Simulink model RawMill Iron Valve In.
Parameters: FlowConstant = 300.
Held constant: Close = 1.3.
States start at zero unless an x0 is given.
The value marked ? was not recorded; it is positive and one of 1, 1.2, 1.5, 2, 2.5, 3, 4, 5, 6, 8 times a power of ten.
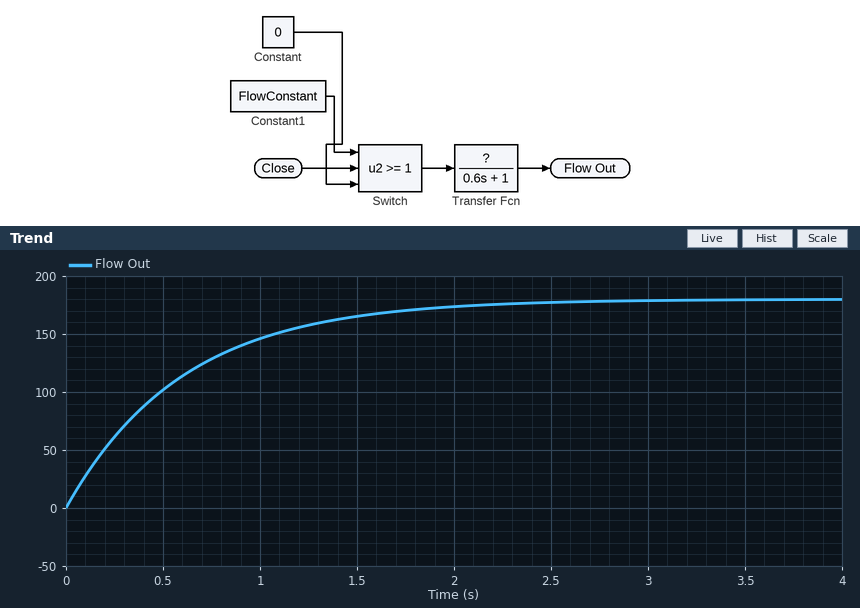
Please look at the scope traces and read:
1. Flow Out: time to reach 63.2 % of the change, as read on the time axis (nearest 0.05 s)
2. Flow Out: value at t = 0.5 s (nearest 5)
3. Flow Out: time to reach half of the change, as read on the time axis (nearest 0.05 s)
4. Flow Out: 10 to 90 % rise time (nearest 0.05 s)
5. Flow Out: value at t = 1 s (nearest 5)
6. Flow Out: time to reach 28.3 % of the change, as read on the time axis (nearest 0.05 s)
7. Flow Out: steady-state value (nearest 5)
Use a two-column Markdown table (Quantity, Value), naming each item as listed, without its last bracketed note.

| Quantity | Value |
|---|---|
| Flow Out: time to reach 63.2 % of the change, as read on the time axis | 0.60 s |
| Flow Out: value at t = 0.5 s | 100 |
| Flow Out: time to reach half of the change, as read on the time axis | 0.40 s |
| Flow Out: 10 to 90 % rise time | 1.30 s |
| Flow Out: value at t = 1 s | 145 |
| Flow Out: time to reach 28.3 % of the change, as read on the time axis | 0.20 s |
| Flow Out: steady-state value | 180 |
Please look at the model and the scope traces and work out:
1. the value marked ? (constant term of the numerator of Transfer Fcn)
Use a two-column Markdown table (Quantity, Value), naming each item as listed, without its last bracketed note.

| Quantity | Value |
|---|---|
| the value marked ? | 0.6 |
